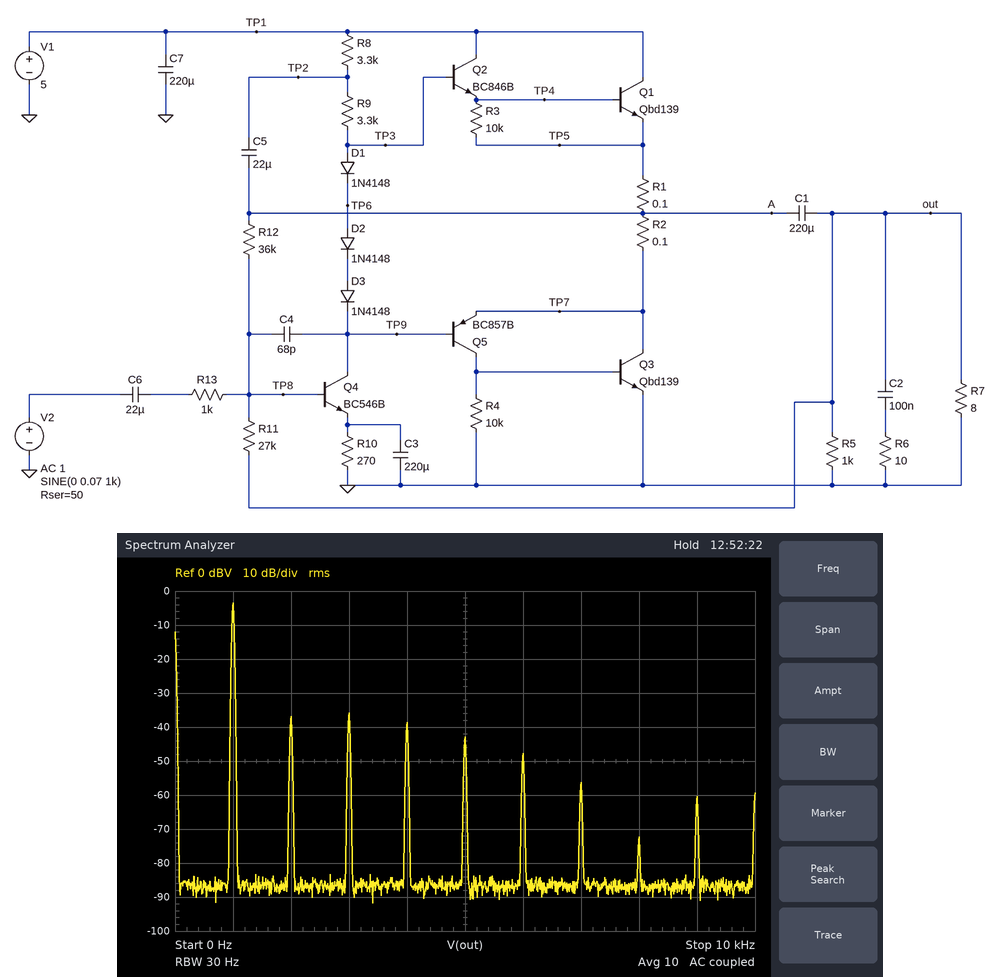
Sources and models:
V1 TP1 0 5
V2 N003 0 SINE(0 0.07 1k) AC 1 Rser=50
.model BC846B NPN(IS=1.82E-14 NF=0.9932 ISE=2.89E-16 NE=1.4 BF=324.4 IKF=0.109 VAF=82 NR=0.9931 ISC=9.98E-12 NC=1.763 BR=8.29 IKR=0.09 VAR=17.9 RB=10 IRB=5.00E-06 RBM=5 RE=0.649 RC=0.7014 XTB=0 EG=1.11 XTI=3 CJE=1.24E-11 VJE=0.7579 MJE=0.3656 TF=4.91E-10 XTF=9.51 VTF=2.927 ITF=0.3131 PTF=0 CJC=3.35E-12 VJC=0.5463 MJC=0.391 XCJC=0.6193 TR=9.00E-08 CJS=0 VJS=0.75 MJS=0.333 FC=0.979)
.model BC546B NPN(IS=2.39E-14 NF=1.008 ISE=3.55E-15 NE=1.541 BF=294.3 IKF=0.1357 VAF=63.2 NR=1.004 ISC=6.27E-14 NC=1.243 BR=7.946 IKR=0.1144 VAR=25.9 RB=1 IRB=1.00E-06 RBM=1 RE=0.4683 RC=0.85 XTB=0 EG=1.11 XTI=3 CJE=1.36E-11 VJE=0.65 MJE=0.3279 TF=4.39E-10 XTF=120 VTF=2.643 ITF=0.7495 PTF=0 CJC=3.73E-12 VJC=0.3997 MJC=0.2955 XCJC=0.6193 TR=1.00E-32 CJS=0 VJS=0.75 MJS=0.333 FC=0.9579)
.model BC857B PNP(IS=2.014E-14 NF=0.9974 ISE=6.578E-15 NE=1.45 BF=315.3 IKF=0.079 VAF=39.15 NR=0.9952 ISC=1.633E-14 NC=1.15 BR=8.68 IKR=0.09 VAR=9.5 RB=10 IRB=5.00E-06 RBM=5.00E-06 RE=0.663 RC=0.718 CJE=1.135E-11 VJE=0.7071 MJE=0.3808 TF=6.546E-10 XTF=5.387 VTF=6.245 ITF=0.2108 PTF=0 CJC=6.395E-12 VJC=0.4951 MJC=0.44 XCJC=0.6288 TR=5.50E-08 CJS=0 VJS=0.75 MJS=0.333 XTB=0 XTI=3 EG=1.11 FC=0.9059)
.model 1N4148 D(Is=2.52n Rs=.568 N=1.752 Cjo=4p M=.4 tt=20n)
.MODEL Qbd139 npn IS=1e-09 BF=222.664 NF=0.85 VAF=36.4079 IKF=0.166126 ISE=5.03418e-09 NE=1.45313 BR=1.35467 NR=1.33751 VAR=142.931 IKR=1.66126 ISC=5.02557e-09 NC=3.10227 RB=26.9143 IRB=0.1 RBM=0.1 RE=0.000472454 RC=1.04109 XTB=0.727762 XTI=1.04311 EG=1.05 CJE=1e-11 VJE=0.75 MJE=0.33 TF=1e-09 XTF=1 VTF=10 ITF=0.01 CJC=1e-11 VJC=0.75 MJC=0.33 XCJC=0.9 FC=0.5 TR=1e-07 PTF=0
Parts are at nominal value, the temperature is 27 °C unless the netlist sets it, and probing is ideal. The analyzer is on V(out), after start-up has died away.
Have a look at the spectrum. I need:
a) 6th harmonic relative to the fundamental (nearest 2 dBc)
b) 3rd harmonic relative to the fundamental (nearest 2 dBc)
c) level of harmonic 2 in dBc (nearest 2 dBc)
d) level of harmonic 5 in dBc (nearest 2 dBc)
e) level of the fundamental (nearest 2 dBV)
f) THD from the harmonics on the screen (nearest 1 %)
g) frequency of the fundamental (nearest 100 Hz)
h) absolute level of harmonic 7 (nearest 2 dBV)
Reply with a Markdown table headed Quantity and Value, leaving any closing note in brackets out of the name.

| Quantity | Value |
|---|---|
| 6th harmonic relative to the fundamental | -44 dBc |
| 3rd harmonic relative to the fundamental | -32 dBc |
| level of harmonic 2 in dBc | -34 dBc |
| level of harmonic 5 in dBc | -40 dBc |
| level of the fundamental | -4 dBV |
| THD from the harmonics on the screen | 4 % |
| frequency of the fundamental | 1.0 kHz |
| absolute level of harmonic 7 | -56 dBV |
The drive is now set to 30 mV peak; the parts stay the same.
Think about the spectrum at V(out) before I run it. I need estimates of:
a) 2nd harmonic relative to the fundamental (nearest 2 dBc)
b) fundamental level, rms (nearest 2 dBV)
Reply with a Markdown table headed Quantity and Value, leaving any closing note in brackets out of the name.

| Quantity | Value |
|---|---|
| 2nd harmonic relative to the fundamental | -50 dBc |
| fundamental level, rms | -10 dBV |
